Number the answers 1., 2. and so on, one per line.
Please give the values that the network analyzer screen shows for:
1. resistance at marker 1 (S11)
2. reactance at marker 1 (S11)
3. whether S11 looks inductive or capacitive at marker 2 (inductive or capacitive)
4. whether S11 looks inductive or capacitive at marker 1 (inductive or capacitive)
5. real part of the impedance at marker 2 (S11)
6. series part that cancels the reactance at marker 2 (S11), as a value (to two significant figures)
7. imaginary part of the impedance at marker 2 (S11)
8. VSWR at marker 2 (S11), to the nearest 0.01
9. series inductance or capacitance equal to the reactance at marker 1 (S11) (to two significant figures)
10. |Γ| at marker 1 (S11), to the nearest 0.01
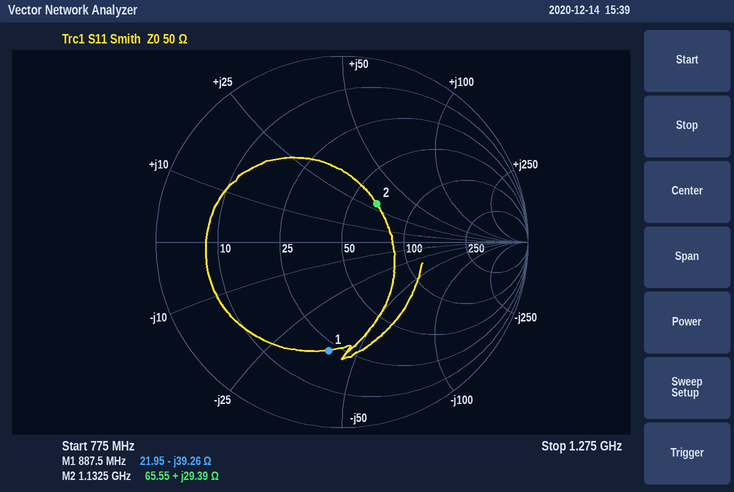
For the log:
1. 21.95 Ω
2. -39.26 Ω
3. inductive
4. capacitive
5. 65.55 Ω
6. 4.8 pF
7. +29.39 Ω
8. 1.77
9. 4.6 pF
10. 0.59
